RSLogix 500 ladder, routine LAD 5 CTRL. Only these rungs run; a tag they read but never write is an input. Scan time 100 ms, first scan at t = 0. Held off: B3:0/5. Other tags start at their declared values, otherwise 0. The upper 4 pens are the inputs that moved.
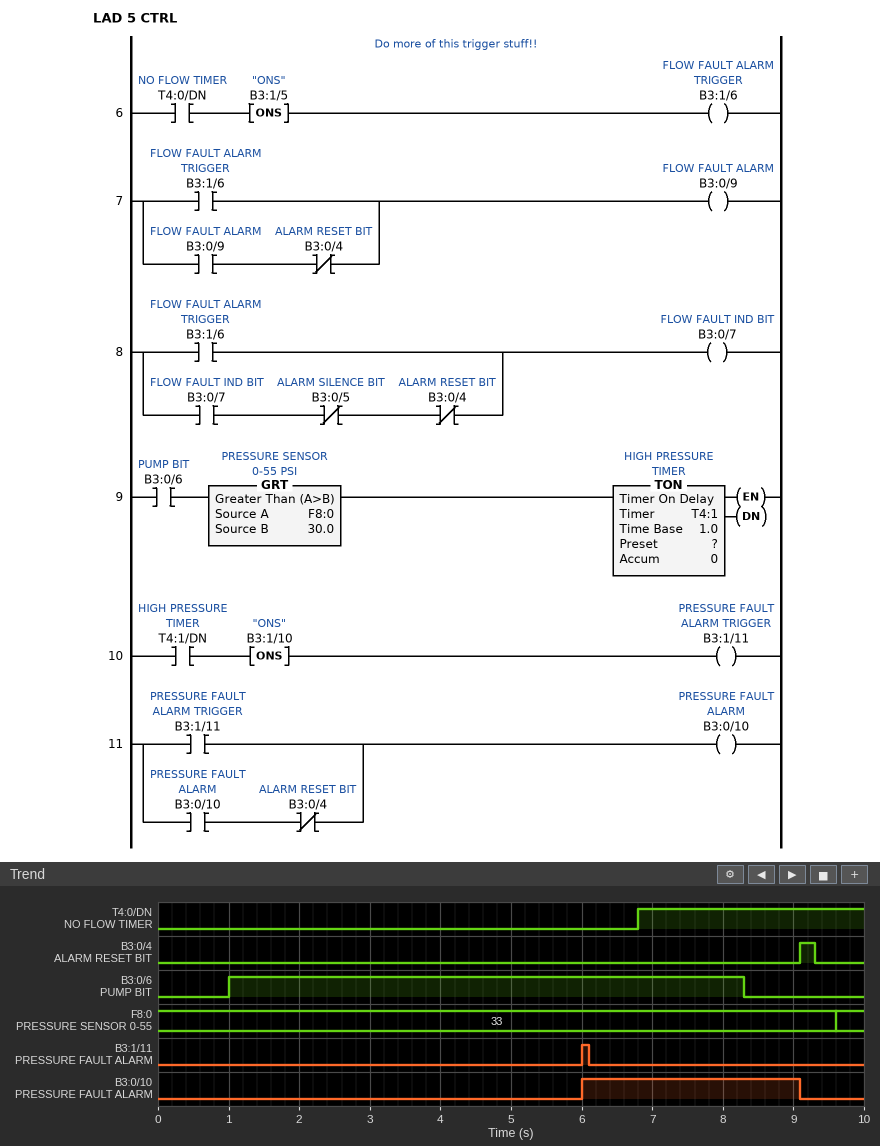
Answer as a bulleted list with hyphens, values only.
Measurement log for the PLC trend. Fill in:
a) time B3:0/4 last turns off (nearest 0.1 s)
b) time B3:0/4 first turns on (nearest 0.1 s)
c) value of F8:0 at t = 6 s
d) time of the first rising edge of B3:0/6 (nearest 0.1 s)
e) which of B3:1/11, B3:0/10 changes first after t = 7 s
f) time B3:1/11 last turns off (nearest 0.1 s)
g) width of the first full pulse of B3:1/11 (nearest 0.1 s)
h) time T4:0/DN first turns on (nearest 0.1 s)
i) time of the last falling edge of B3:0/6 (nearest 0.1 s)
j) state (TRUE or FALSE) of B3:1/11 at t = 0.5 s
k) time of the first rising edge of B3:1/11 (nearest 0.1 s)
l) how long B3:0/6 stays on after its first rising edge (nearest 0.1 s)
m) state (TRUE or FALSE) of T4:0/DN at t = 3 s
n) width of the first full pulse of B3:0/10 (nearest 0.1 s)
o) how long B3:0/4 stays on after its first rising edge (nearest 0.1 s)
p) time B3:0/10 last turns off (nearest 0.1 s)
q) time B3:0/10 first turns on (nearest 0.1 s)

- 9.3 s
- 9.1 s
- 33
- 1.0 s
- B3:0/10
- 6.1 s
- 0.1 s
- 6.8 s
- 8.3 s
- FALSE
- 6.0 s
- 7.3 s
- FALSE
- 3.1 s
- 0.2 s
- 9.1 s
- 6.0 s
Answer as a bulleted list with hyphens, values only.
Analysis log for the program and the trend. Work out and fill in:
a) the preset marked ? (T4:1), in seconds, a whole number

- 5 s
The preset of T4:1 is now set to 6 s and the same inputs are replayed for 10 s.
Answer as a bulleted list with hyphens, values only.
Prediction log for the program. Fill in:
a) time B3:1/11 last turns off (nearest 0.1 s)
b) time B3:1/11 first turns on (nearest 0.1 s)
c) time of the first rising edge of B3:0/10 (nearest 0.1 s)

- 7.1 s
- 7.0 s
- 7.0 s
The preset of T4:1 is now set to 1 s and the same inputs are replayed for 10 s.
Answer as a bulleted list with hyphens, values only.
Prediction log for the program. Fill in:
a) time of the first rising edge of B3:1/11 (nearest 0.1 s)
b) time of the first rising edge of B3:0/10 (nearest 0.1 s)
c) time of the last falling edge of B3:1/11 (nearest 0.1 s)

- 2.0 s
- 2.0 s
- 2.1 s
